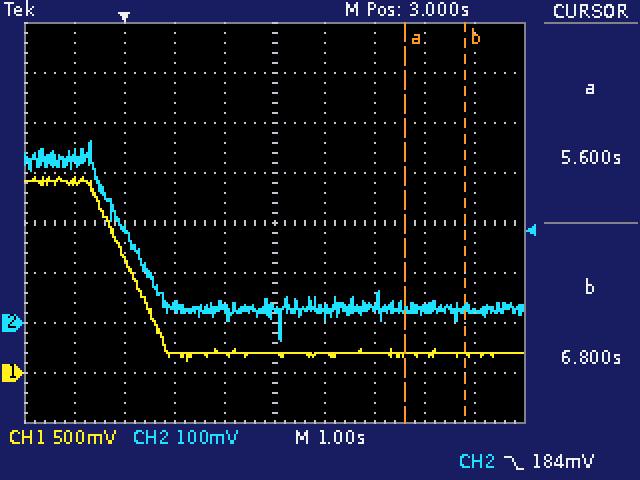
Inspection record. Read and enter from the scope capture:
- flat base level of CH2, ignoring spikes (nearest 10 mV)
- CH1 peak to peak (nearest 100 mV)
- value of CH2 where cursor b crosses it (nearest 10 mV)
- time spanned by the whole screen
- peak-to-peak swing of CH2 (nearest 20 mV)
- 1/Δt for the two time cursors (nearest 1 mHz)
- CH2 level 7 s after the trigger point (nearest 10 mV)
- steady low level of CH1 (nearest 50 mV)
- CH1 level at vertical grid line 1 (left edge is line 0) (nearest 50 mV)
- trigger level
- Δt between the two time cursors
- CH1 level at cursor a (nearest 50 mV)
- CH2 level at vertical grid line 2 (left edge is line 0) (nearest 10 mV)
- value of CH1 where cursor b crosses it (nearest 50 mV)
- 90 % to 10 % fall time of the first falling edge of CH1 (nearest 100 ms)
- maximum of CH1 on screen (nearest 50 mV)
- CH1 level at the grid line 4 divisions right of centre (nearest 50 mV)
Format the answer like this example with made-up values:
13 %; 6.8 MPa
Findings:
30 mV; 1.80 V; 30 mV; 10 s; 400 mV; 833 mHz; 20 mV; 200 mV; 1.90 V; 184 mV; 1.2 s; 200 mV; 190 mV; 200 mV; 1.3 s; 1.95 V; 200 mV
